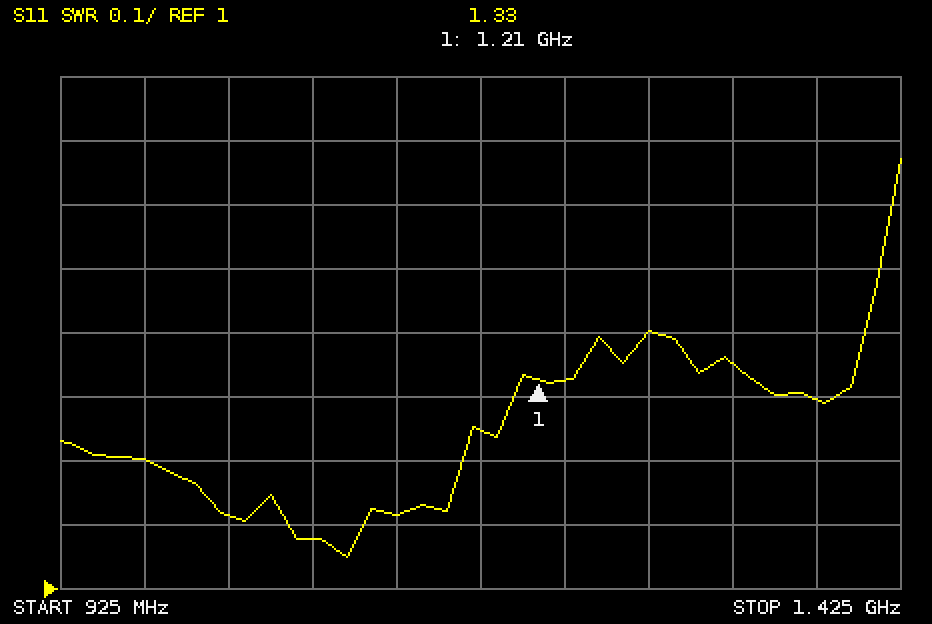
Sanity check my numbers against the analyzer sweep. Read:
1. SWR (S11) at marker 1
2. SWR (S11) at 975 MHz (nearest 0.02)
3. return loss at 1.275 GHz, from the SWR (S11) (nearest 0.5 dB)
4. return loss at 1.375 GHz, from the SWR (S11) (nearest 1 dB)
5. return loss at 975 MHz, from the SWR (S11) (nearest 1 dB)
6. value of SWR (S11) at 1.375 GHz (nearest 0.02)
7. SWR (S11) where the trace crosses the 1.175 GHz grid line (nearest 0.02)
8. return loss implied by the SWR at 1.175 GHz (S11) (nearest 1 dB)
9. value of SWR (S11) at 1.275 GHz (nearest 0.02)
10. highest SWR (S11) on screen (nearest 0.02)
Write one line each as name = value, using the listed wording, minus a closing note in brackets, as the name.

SWR (S11) at marker 1 = 1.33
SWR (S11) at 975 MHz = 1.20
return loss at 1.275 GHz, from the SWR (S11) = 15.5 dB
return loss at 1.375 GHz, from the SWR (S11) = 18 dB
return loss at 975 MHz, from the SWR (S11) = 21 dB
value of SWR (S11) at 1.375 GHz = 1.30
SWR (S11) where the trace crosses the 1.175 GHz grid line = 1.24
return loss implied by the SWR at 1.175 GHz (S11) = 19 dB
value of SWR (S11) at 1.275 GHz = 1.40
highest SWR (S11) on screen = 1.68
